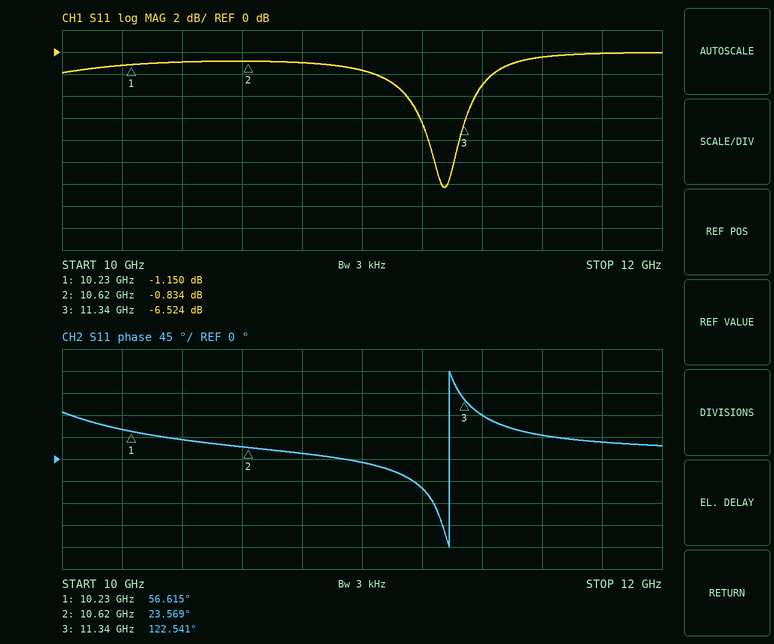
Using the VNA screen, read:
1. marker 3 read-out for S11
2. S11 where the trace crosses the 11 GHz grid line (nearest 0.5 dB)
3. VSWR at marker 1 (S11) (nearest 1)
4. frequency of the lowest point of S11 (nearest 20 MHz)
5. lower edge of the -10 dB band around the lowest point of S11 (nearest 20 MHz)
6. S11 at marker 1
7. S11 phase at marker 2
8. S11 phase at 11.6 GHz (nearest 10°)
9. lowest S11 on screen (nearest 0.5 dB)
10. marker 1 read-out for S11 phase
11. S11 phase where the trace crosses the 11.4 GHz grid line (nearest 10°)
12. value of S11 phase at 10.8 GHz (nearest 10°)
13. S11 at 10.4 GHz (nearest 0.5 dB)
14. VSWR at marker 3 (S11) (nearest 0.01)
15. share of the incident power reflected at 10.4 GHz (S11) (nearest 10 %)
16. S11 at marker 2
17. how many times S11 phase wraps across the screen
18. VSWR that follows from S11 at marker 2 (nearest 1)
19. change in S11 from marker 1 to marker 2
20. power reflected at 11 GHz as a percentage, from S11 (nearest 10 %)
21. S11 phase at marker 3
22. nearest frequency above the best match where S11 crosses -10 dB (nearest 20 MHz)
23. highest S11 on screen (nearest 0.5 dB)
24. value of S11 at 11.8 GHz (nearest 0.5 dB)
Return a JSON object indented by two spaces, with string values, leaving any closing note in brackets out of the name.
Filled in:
{
  "marker 3 read-out for S11": "-6.524 dB",
  "S11 where the trace crosses the 11 GHz grid line": "-1.5 dB",
  "VSWR at marker 1 (S11)": "15",
  "frequency of the lowest point of S11": "11.28 GHz",
  "lower edge of the -10 dB band around the lowest point of S11": "11.24 GHz",
  "S11 at marker 1": "-1.150 dB",
  "S11 phase at marker 2": "23.569°",
  "S11 phase at 11.6 GHz": "50°",
  "lowest S11 on screen": "-12.5 dB",
  "marker 1 read-out for S11 phase": "56.615°",
  "S11 phase where the trace crosses the 11.4 GHz grid line": "90°",
  "value of S11 phase at 10.8 GHz": "10°",
  "S11 at 10.4 GHz": "-1.0 dB",
  "VSWR at marker 3 (S11)": "2.79",
  "share of the incident power reflected at 10.4 GHz (S11)": "80 %",
  "S11 at marker 2": "-0.834 dB",
  "how many times S11 phase wraps across the screen": "1",
  "VSWR that follows from S11 at marker 2": "21",
  "change in S11 from marker 1 to marker 2": "0.316 dB",
  "power reflected at 11 GHz as a percentage, from S11": "70 %",
  "S11 phase at marker 3": "122.541°",
  "nearest frequency above the best match where S11 crosses -10 dB": "11.30 GHz",
  "highest S11 on screen": "0.0 dB",
  "value of S11 at 11.8 GHz": "0.0 dB"
}
